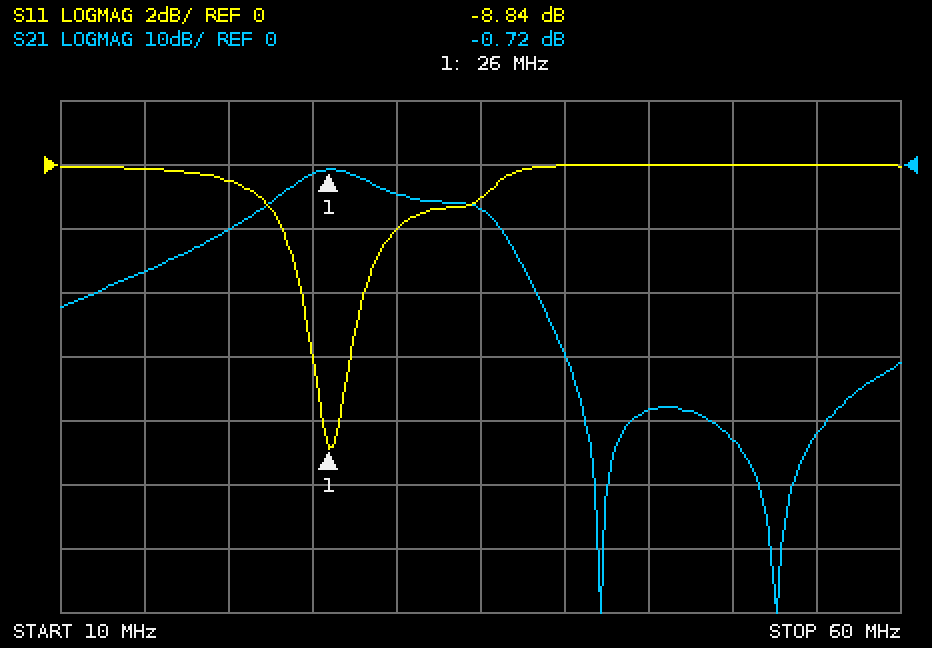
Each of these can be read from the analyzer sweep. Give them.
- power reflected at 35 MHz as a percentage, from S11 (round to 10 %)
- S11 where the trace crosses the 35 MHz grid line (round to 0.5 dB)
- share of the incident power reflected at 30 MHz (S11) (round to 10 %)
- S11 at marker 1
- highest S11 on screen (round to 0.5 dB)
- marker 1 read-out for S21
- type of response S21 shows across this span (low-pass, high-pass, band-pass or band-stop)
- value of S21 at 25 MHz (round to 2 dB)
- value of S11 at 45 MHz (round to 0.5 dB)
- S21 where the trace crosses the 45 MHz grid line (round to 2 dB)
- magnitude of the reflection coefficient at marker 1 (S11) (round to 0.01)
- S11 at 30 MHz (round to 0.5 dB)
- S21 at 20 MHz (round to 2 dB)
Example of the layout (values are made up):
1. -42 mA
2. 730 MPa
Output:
1. 80 %
2. -1.0 dB
3. 60 %
4. -8.84 dB
5. 0.0 dB
6. -0.72 dB
7. band-pass
8. -2 dB
9. 0.0 dB
10. -38 dB
11. 0.36
12. -2.0 dB
13. -10 dB
